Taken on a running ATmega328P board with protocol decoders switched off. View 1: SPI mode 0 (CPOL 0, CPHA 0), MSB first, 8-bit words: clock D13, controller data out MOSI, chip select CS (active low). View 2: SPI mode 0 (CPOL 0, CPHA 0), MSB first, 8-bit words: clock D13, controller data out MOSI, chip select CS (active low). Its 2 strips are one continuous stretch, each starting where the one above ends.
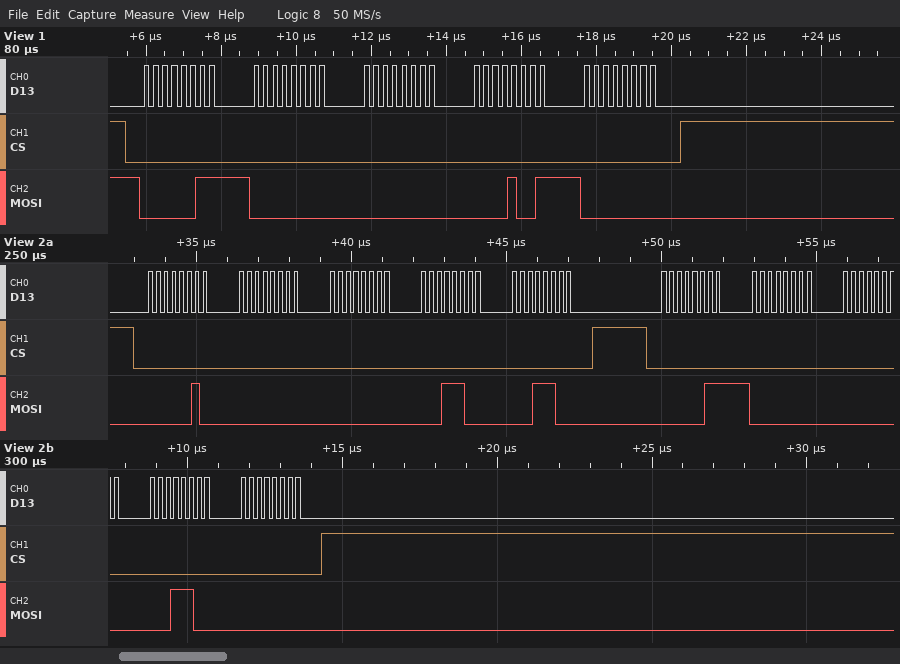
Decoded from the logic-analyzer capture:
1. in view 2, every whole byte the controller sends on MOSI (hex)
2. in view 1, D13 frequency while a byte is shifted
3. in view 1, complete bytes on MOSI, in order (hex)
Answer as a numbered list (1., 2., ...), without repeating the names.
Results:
1. 0x02 0x00 0x00 0x1C 0x1C 0x03 0x00 0x00 0x1C 0x00
2. 4 MHz
3. 03 00 00 09 00
